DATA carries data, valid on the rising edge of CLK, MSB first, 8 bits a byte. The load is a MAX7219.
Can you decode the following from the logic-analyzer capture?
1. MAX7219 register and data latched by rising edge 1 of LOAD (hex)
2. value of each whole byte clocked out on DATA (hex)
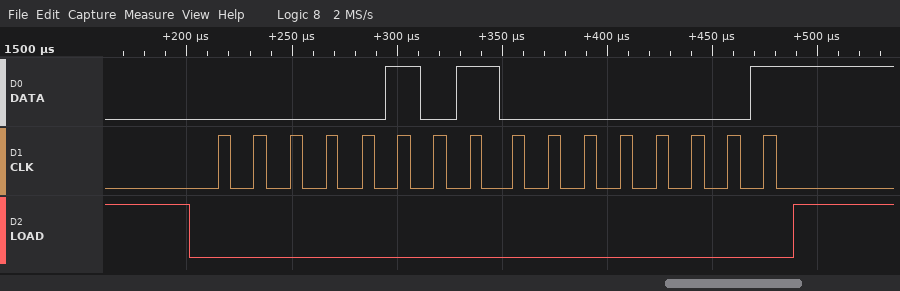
register 0x5, data 0x01
05 01
